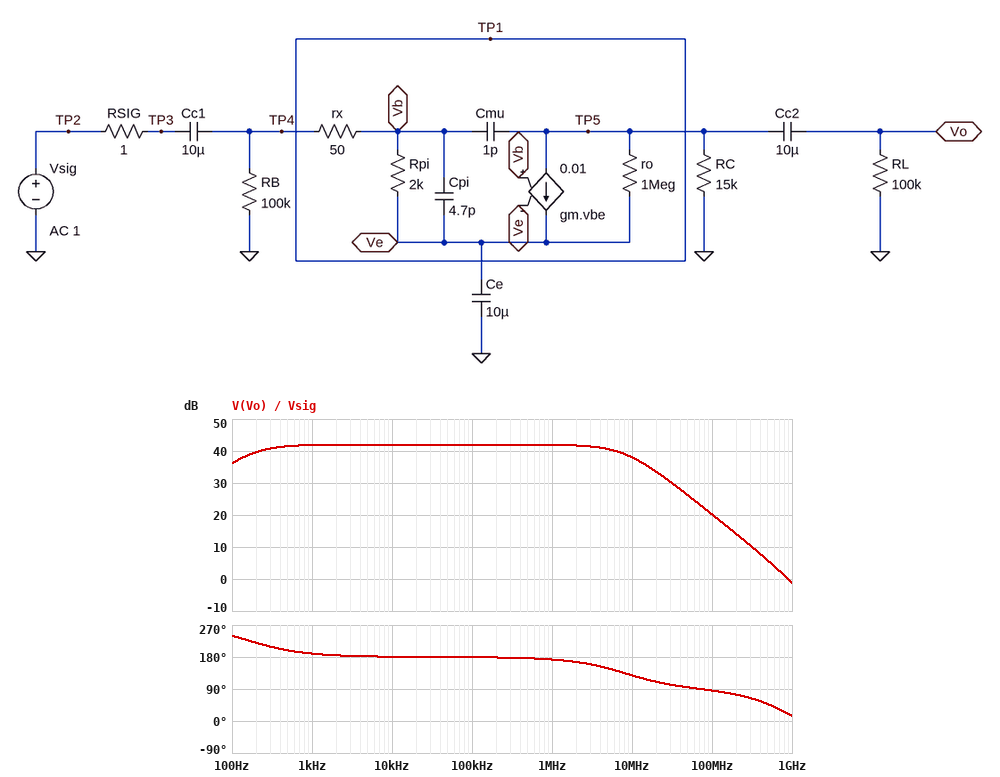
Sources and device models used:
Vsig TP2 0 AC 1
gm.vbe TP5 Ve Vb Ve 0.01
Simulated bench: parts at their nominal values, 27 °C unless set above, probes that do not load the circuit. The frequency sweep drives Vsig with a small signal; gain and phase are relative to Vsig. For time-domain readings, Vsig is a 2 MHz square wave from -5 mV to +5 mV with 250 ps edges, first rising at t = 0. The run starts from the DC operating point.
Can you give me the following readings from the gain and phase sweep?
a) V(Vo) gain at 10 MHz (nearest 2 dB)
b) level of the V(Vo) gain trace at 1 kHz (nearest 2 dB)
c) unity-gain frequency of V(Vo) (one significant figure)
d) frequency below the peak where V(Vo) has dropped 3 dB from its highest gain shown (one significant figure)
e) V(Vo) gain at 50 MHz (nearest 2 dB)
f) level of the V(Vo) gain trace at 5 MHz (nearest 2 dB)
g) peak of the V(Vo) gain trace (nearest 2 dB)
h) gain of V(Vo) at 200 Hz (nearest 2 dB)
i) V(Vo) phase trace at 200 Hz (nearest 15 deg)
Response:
38 dB
42 dB
900 MHz
200 Hz
26 dB
40 dB
42 dB
40 dB
225 deg
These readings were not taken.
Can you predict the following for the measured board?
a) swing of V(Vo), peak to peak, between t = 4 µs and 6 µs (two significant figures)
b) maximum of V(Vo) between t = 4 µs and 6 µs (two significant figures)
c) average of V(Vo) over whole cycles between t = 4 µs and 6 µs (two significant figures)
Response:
1.3 V
4.5 mV
-620 mV
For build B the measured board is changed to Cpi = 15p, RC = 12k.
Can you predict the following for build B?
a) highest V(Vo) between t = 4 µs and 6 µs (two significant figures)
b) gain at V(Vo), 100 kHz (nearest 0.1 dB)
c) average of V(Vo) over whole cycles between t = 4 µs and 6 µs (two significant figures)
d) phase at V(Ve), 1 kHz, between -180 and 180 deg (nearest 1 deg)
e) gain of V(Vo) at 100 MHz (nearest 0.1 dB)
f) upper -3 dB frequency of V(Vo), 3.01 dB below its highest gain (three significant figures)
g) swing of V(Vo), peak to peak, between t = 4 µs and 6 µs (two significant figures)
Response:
3.5 mV
40.3 dB
-510 mV
-80 deg
19.7 dB
9.83 MHz
1.0 V
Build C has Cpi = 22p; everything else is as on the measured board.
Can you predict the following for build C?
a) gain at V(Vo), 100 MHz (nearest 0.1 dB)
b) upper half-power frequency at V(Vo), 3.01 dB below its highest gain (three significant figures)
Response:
19.3 dB
8.07 MHz
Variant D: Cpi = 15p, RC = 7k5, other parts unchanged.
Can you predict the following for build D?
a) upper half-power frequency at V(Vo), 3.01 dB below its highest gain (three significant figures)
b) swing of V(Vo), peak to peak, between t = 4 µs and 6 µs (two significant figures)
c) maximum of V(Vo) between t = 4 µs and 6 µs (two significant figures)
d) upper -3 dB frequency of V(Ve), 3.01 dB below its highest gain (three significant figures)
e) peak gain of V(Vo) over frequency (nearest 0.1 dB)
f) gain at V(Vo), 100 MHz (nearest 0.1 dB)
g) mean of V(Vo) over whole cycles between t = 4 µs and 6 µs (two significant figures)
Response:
14.9 MHz
680 mV
2.4 mV
170 Hz
36.6 dB
19.6 dB
-340 mV
